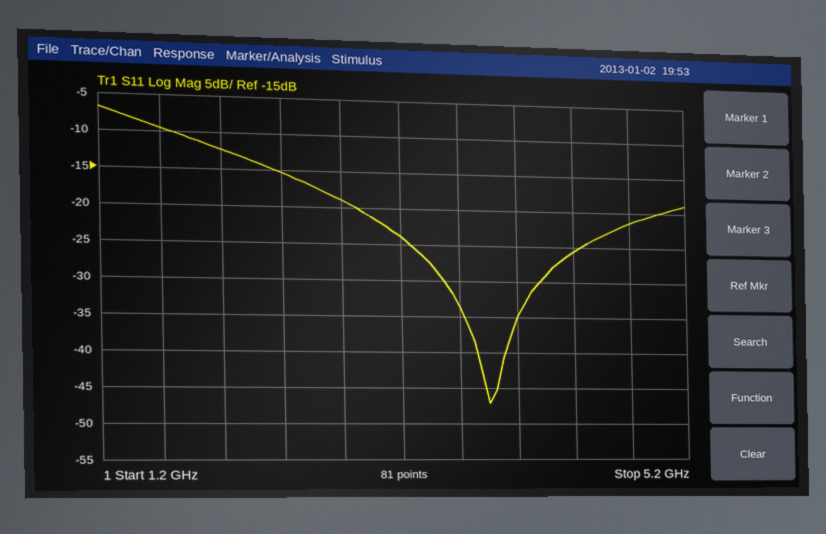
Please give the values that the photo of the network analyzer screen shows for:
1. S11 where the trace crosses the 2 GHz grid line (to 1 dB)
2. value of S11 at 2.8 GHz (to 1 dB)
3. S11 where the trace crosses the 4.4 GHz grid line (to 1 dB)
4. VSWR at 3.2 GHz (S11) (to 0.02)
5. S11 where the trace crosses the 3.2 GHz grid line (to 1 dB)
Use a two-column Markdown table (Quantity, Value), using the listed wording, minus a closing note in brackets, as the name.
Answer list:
| Quantity | Value |
|---|---|
| S11 where the trace crosses the 2 GHz grid line | -12 dB |
| value of S11 at 2.8 GHz | -19 dB |
| S11 where the trace crosses the 4.4 GHz grid line | -26 dB |
| VSWR at 3.2 GHz (S11) | 1.14 |
| S11 where the trace crosses the 3.2 GHz grid line | -24 dB |
